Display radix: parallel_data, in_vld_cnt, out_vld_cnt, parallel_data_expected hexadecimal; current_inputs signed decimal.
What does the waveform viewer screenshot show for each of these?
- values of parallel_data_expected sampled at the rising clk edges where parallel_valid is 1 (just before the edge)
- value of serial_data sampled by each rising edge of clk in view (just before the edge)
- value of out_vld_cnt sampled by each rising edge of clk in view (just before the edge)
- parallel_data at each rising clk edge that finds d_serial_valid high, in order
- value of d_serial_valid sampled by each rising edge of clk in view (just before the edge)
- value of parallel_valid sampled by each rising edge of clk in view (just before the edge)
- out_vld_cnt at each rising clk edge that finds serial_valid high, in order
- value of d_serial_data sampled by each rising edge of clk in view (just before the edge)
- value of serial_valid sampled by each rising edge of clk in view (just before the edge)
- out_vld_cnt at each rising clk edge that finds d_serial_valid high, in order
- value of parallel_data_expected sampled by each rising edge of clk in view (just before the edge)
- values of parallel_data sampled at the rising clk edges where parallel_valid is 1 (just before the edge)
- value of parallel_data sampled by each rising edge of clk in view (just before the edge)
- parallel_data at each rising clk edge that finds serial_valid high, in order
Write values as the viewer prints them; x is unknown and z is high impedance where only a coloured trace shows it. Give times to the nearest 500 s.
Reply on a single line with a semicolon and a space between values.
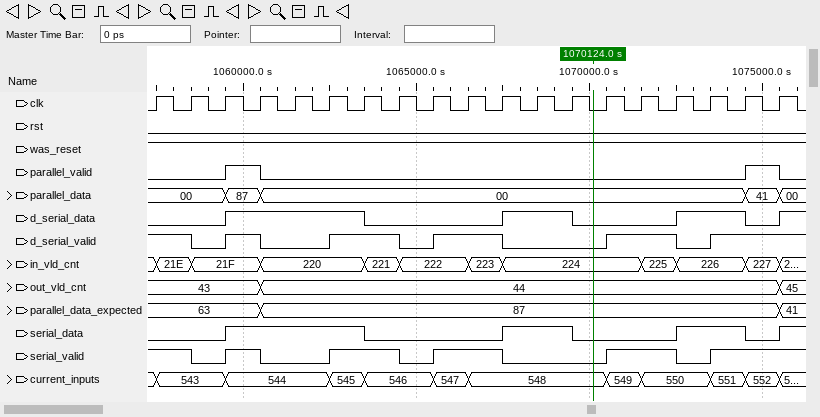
63, 87; 0 0 0 1 1 1 1 0 0 0 0 1 1 0 0 0 1 1 0; 43, 43, 43, 43, 44, 44, 44, 44, 44, 44, 44, 44, 44, 44, 44, 44, 44, 44, 44; 00, 00, 87, 00, 00, 00, 00, 00, 00, 00, 41; 1 1 0 1 0 0 1 1 0 1 1 0 0 0 1 1 0 1 1; 0 0 0 1 0 0 0 0 0 0 0 0 0 0 0 0 0 0 1; 43, 43, 43, 44, 44, 44, 44, 44, 44, 44, 44; 0 0 0 1 1 1 1 0 0 0 0 1 1 0 0 0 1 1 0; 1 1 0 1 0 0 1 1 0 1 1 0 0 0 1 1 0 1 1; 43, 43, 43, 44, 44, 44, 44, 44, 44, 44, 44; 63, 63, 63, 63, 87, 87, 87, 87, 87, 87, 87, 87, 87, 87, 87, 87, 87, 87, 87; 87, 41; 00, 00, 00, 87, 00, 00, 00, 00, 00, 00, 00, 00, 00, 00, 00, 00, 00, 00, 41; 00, 00, 87, 00, 00, 00, 00, 00, 00, 00, 41
